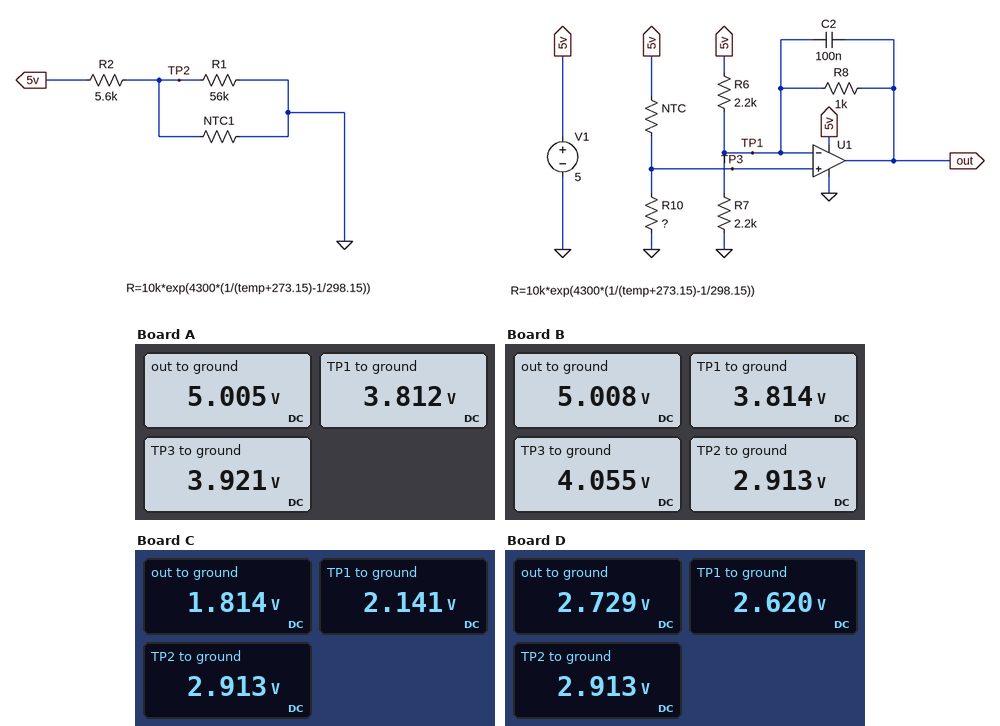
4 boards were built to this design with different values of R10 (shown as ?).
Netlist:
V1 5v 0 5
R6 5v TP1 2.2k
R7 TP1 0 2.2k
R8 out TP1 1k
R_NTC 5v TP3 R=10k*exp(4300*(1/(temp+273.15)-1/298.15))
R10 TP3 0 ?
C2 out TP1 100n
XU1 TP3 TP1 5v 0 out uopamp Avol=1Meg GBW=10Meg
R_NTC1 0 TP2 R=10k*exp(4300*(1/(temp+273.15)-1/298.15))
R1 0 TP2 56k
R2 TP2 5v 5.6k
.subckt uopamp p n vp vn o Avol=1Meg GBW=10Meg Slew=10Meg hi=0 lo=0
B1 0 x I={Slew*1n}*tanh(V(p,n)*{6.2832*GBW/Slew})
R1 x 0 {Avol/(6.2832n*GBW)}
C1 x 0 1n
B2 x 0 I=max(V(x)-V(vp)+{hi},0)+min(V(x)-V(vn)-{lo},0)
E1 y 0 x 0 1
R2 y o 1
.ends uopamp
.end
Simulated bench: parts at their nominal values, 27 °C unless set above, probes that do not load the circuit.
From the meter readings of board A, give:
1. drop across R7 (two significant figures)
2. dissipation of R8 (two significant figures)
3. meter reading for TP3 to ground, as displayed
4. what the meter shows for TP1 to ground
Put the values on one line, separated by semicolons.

3.8 V; 1.4 mW; 3.921 V; 3.812 V
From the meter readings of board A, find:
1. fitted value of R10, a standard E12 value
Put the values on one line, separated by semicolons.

33 kΩ
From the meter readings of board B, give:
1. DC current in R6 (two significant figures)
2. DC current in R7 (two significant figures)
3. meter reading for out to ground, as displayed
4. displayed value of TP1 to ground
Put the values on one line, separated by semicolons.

540 µA; 1.7 mA; 5.008 V; 3.814 V
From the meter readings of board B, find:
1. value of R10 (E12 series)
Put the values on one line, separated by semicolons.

39 kΩ
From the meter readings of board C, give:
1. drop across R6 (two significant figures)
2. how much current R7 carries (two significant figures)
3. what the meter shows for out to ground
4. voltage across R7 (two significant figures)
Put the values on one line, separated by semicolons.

2.9 V; 970 µA; 1.814 V; 2.1 V
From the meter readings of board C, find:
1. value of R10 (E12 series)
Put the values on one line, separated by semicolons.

6.8 kΩ
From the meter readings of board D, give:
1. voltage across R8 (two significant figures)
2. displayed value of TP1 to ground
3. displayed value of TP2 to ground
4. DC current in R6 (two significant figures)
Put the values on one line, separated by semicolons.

110 mV; 2.620 V; 2.913 V; 1.1 mA
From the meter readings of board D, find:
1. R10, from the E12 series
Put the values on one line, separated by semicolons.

10 kΩ
